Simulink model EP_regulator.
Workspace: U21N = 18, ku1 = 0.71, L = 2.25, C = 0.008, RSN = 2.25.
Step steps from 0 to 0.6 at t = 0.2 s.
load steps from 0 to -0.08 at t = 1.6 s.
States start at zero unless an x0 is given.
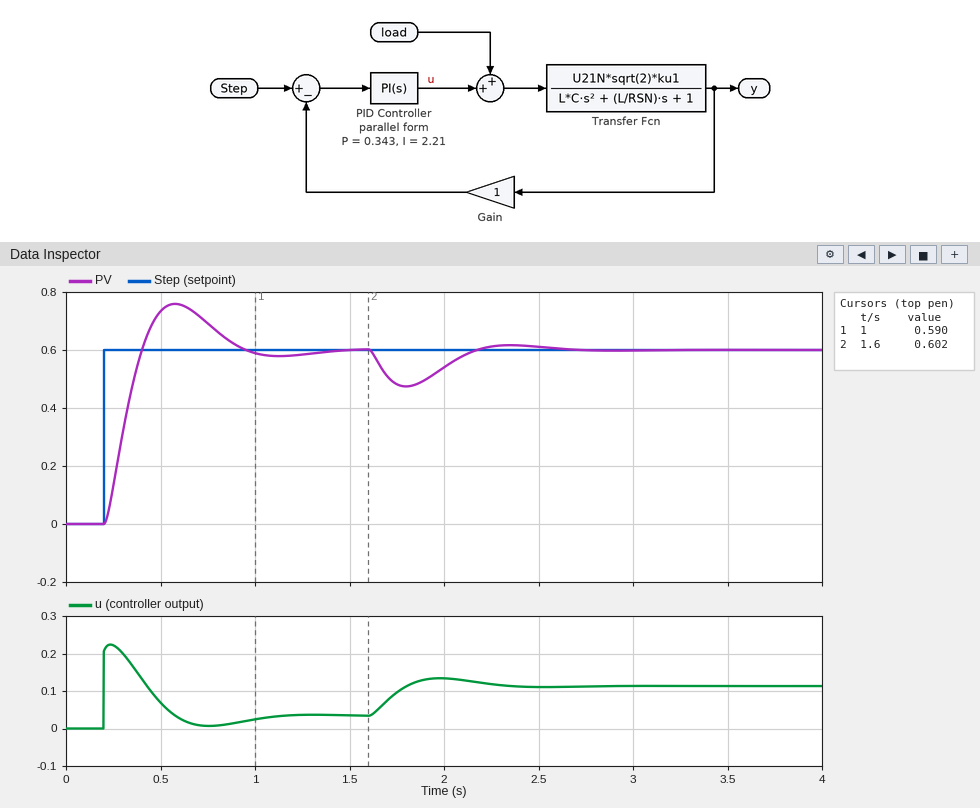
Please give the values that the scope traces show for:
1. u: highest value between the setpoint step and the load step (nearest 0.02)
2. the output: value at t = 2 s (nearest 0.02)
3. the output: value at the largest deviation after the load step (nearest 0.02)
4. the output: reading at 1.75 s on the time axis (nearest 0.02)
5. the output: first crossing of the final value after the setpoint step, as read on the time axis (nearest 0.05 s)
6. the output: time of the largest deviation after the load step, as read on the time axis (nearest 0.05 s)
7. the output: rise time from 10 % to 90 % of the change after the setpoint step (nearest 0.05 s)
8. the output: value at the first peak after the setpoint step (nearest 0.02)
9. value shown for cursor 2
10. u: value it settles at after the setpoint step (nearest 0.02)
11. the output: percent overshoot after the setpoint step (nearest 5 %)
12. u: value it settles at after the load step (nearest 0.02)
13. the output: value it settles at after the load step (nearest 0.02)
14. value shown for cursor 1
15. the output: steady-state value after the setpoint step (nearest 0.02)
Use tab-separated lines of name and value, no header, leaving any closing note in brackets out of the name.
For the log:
u: highest value between the setpoint step and the load step	0.22
the output: value at t = 2 s	0.54
the output: value at the largest deviation after the load step	0.48
the output: reading at 1.75 s on the time axis	0.48
the output: first crossing of the final value after the setpoint step, as read on the time axis	0.40 s
the output: time of the largest deviation after the load step, as read on the time axis	1.80 s
the output: rise time from 10 % to 90 % of the change after the setpoint step	0.15 s
the output: value at the first peak after the setpoint step	0.76
value shown for cursor 2	0.602
u: value it settles at after the setpoint step	0.04
the output: percent overshoot after the setpoint step	25 %
u: value it settles at after the load step	0.12
the output: value it settles at after the load step	0.60
value shown for cursor 1	0.590
the output: steady-state value after the setpoint step	0.60
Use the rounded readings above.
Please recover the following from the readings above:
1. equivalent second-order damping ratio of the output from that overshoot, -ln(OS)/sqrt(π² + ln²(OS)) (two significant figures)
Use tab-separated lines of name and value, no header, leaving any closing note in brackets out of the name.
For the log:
equivalent second-order damping ratio of the output from that overshoot, -ln(OS)/sqrt(π² + ln²(OS))	0.40
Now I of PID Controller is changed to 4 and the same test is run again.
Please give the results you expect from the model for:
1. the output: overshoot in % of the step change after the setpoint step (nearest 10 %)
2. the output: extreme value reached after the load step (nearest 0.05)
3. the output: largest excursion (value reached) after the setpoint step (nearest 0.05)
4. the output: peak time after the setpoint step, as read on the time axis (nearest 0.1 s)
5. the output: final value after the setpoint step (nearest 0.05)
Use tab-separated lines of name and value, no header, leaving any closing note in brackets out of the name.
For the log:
the output: overshoot in % of the step change after the setpoint step	40 %
the output: extreme value reached after the load step	0.50
the output: largest excursion (value reached) after the setpoint step	0.85
the output: peak time after the setpoint step, as read on the time axis	0.5 s
the output: final value after the setpoint step	0.60
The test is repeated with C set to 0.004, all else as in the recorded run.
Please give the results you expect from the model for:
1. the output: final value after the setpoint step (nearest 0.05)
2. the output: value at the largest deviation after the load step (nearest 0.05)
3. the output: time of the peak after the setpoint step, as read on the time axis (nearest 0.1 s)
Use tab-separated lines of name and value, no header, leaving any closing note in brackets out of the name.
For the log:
the output: final value after the setpoint step	0.60
the output: value at the largest deviation after the load step	0.50
the output: time of the peak after the setpoint step, as read on the time axis	0.6 s
